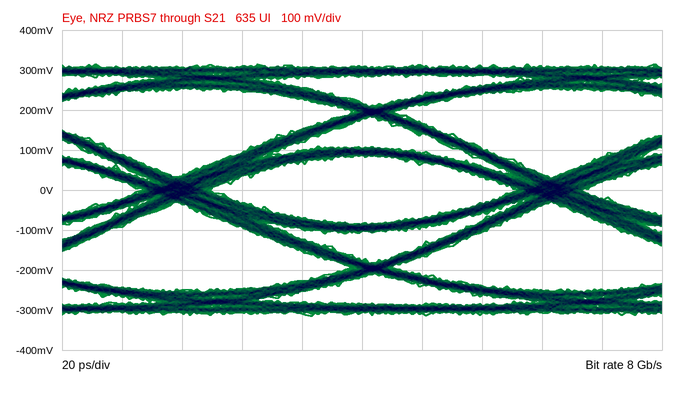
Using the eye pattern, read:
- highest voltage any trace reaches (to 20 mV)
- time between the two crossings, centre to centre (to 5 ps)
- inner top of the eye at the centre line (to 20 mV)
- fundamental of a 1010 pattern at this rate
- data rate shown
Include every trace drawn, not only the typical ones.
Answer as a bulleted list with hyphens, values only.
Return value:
- 320 mV
- 125 ps
- 80 mV
- 4 GHz
- 8 Gb/s
